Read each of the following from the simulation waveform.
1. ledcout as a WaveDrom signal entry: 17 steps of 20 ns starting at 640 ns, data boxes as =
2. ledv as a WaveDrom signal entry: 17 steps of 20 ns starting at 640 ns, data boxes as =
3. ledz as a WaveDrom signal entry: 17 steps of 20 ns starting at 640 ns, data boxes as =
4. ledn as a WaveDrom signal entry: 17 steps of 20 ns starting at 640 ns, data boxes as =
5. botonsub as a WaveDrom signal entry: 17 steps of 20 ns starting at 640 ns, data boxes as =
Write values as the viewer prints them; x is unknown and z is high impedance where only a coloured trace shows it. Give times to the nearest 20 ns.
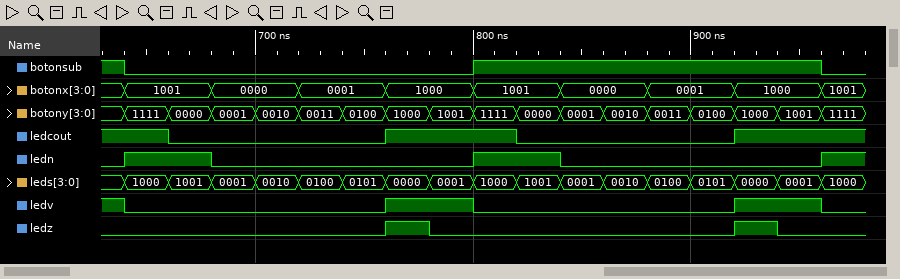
{name: 'ledcout', wave: '10....1..0....1..'}
{name: 'ledv', wave: '0.....1.0.....1.0'}
{name: 'ledz', wave: '0.....10......10.'}
{name: 'ledn', wave: '1.0.....1.0.....1'}
{name: 'botonsub', wave: '0.......1.......0'}
